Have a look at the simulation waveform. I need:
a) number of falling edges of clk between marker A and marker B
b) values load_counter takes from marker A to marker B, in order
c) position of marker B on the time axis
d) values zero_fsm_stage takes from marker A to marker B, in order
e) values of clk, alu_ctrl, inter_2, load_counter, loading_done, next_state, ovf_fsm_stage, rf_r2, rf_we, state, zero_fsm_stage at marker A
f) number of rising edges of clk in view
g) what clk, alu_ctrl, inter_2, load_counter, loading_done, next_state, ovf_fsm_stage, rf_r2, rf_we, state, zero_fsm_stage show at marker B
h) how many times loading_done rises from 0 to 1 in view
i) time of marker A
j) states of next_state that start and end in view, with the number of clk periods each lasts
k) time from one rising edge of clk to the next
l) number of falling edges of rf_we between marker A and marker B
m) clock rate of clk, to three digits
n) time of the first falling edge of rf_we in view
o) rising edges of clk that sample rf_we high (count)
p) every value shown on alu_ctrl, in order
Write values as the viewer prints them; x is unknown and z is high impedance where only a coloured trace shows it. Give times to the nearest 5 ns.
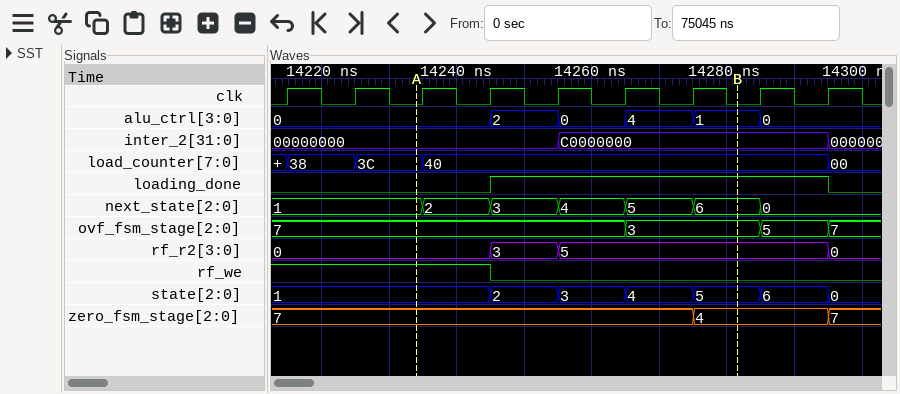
5
3C, 40
14280 ns
7, 4
clk=0, alu_ctrl=0, inter_2=00000000, load_counter=3C, loading_done=0, next_state=1, ovf_fsm_stage=7, rf_r2=0, rf_we=1, state=1, zero_fsm_stage=7
9
clk=0, alu_ctrl=1, inter_2=C0000000, load_counter=40, loading_done=1, next_state=6, ovf_fsm_stage=3, rf_r2=5, rf_we=0, state=5, zero_fsm_stage=4
1
14235 ns
2: 1, 3: 1, 4: 1, 5: 1, 6: 1
10 ns
1
100 MHz
14245 ns
4
0, 2, 0, 4, 1, 0
